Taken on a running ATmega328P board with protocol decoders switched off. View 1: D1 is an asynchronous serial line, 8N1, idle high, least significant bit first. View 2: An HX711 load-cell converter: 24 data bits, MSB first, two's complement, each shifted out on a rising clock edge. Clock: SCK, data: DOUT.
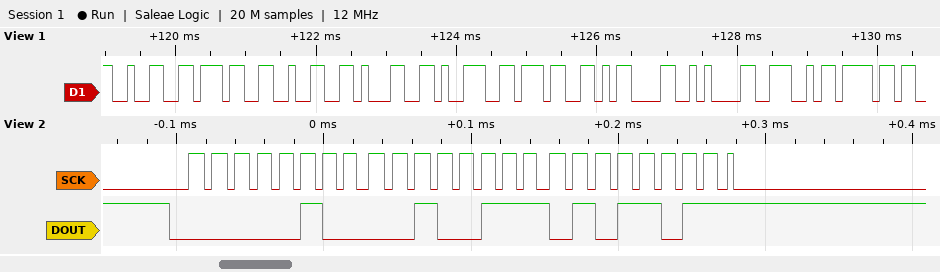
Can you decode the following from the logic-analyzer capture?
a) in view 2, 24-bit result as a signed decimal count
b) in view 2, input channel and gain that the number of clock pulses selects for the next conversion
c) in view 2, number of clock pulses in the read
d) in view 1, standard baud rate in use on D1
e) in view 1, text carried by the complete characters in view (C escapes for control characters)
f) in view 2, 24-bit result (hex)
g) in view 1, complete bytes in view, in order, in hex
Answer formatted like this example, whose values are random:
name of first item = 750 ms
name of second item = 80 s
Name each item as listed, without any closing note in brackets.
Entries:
in view 2, 24-bit result as a signed decimal count = 272219
in view 2, input channel and gain that the number of clock pulses selects for the next conversion = channel A, gain 128
in view 2, number of clock pulses in the read = 25
in view 1, standard baud rate in use on D1 = 9600 baud
in view 1, text carried by the complete characters in view = "272197\r\nNo"
in view 2, 24-bit result = 0x04275B
in view 1, complete bytes in view, in order, in hex = 32 37 32 31 39 37 0D 0A 4E 6F
